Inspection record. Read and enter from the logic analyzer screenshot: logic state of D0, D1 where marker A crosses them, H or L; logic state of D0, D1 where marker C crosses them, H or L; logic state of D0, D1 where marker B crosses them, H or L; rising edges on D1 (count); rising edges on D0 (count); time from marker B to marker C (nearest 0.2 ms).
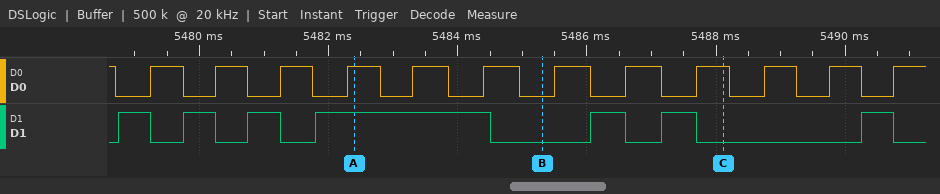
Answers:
D0=H, D1=H
D0=H, D1=L
D0=L, D1=L
7
12
2.8 ms
